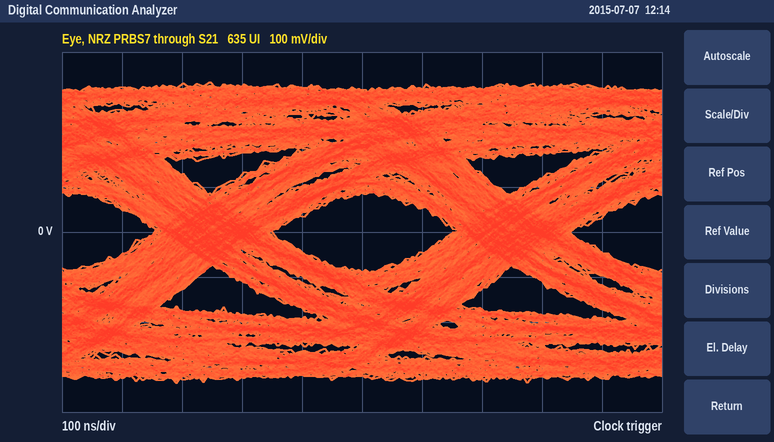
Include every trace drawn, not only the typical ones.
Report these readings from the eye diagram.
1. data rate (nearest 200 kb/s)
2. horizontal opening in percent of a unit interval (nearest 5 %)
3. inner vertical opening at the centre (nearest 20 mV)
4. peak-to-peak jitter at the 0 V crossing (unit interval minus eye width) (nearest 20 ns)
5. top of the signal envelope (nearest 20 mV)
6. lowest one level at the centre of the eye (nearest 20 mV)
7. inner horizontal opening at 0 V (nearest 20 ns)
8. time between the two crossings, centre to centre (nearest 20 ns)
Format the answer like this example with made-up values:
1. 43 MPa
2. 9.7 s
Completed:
1. 2.0 Mb/s
2. 60 %
3. 180 mV
4. 200 ns
5. 340 mV
6. 80 mV
7. 300 ns
8. 500 ns
